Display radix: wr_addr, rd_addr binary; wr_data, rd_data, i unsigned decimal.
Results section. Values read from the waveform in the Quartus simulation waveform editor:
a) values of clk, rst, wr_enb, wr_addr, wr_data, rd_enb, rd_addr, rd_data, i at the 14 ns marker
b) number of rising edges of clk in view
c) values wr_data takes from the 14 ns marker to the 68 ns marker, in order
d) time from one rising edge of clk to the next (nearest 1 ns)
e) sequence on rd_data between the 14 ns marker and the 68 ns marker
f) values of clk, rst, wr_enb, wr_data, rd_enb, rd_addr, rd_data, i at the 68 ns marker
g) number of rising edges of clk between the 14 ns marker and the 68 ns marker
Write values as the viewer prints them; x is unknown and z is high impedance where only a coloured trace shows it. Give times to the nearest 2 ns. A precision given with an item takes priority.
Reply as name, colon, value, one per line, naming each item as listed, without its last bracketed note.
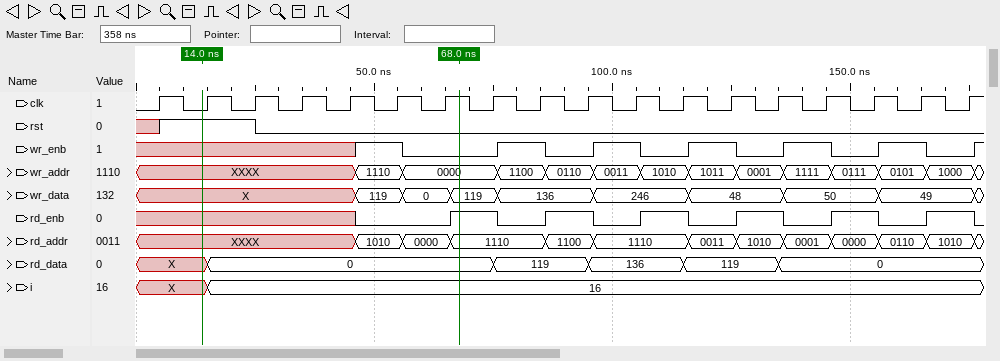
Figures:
values of clk, rst, wr_enb, wr_addr, wr_data, rd_enb, rd_addr, rd_data, i at the 14 ns marker: clk=0, rst=1, wr_enb=x, wr_addr=XXXX, wr_data=X, rd_enb=x, rd_addr=XXXX, rd_data=X, i=X
number of rising edges of clk in view: 18
values wr_data takes from the 14 ns marker to the 68 ns marker, in order: X, 119, 0, 119
time from one rising edge of clk to the next: 10 ns
sequence on rd_data between the 14 ns marker and the 68 ns marker: X, 0
values of clk, rst, wr_enb, wr_data, rd_enb, rd_addr, rd_data, i at the 68 ns marker: clk=1, rst=0, wr_enb=0, wr_data=119, rd_enb=1, rd_addr=1110, rd_data=0, i=16
number of rising edges of clk between the 14 ns marker and the 68 ns marker: 6
